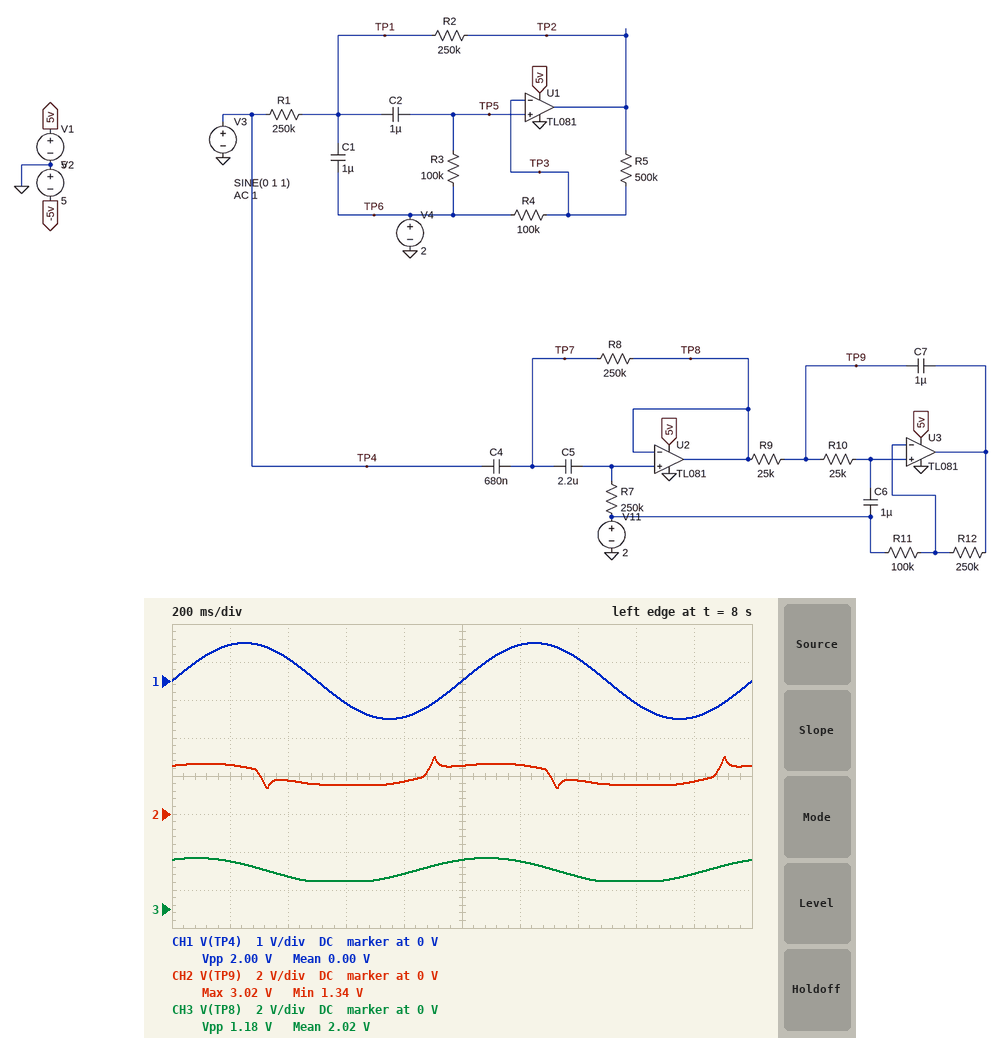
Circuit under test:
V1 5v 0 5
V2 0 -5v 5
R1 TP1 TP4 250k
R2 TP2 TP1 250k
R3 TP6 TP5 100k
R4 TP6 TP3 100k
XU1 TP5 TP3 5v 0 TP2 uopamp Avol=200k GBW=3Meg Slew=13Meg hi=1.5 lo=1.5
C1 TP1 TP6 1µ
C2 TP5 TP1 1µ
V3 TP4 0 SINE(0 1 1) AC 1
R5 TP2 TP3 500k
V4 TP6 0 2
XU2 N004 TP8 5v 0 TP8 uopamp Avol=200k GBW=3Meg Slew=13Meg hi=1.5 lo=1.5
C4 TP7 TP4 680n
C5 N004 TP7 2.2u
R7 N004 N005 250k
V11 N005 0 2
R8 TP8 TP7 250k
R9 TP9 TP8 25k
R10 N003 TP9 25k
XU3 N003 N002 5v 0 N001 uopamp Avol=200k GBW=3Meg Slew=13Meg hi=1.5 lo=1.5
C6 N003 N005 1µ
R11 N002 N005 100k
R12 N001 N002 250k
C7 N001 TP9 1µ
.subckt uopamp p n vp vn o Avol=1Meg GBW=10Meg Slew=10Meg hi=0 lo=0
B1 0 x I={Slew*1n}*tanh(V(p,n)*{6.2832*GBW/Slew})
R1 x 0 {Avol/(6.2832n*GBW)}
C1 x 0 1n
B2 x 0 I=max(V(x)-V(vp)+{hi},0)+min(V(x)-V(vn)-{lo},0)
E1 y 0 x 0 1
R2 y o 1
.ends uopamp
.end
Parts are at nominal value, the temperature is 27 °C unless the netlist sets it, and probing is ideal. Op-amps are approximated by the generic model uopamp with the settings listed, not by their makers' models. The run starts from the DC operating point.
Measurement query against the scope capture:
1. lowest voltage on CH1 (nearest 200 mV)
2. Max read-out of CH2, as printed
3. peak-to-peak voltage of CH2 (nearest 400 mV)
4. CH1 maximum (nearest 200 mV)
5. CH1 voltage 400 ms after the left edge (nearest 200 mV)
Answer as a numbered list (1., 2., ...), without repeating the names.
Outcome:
1. -1.0 V
2. 3.02 V
3. 1.6 V
4. 1.0 V
5. 600 mV
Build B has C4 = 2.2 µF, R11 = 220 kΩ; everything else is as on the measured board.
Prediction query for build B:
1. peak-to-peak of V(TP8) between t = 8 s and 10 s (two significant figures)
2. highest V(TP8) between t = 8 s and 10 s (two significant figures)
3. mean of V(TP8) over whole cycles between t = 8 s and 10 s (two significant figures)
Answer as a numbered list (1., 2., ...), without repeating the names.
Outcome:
1. 1.4 V
2. 2.9 V
3. 2.1 V
